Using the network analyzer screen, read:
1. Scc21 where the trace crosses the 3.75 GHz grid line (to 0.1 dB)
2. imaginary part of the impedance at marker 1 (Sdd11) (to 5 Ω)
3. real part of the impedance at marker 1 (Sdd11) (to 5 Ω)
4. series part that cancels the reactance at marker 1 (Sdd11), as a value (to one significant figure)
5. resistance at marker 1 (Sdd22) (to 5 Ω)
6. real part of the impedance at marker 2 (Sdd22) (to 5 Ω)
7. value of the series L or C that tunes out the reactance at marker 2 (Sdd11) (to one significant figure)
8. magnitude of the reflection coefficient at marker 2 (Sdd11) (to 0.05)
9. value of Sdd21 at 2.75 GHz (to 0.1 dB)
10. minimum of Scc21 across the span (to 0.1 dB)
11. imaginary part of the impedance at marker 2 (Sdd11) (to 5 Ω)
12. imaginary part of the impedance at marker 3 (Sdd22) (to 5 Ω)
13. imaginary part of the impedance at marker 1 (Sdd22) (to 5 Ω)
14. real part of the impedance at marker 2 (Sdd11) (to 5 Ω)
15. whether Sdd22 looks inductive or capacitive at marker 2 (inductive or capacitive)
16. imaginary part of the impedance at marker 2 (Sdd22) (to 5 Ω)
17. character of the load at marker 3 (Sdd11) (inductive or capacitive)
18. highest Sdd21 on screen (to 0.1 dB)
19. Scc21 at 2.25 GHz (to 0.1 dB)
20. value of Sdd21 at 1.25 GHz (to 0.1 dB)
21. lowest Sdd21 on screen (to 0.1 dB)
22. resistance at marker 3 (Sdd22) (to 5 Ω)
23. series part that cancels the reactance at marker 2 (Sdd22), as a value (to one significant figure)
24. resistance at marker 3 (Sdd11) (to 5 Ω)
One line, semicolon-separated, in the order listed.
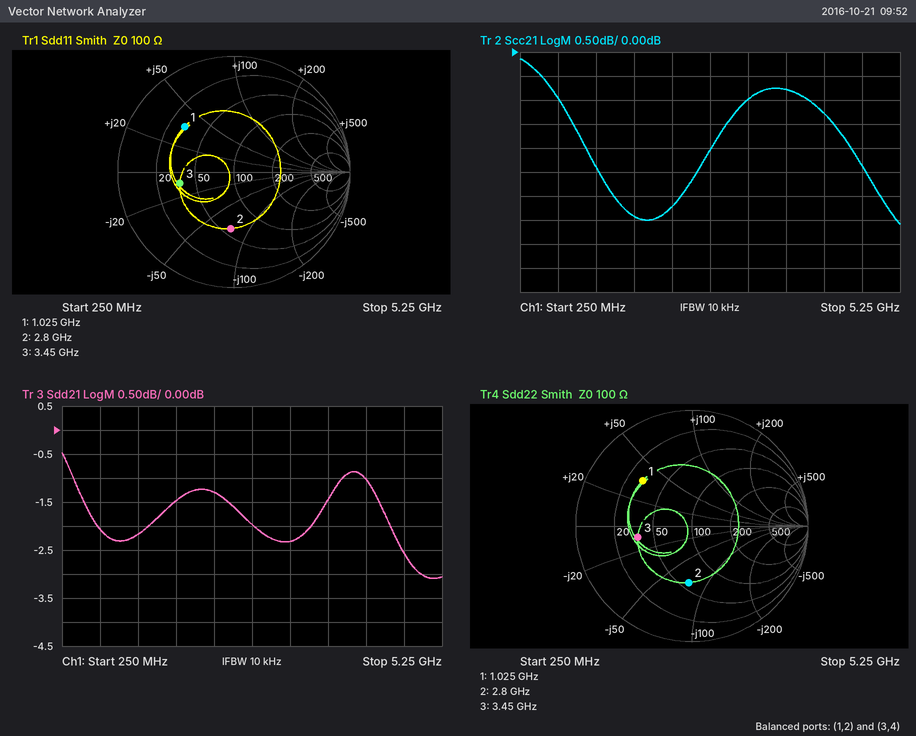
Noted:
-0.8 dB; +35 Ω; 30 Ω; 4 pF; 30 Ω; 60 Ω; 4 nH; 0.50; -2.0 dB; -3.6 dB; -75 Ω; -10 Ω; +35 Ω; 60 Ω; capacitive; -75 Ω; capacitive; -0.5 dB; -3.2 dB; -2.2 dB; -3.1 dB; 35 Ω; 4 nH; 35 Ω
